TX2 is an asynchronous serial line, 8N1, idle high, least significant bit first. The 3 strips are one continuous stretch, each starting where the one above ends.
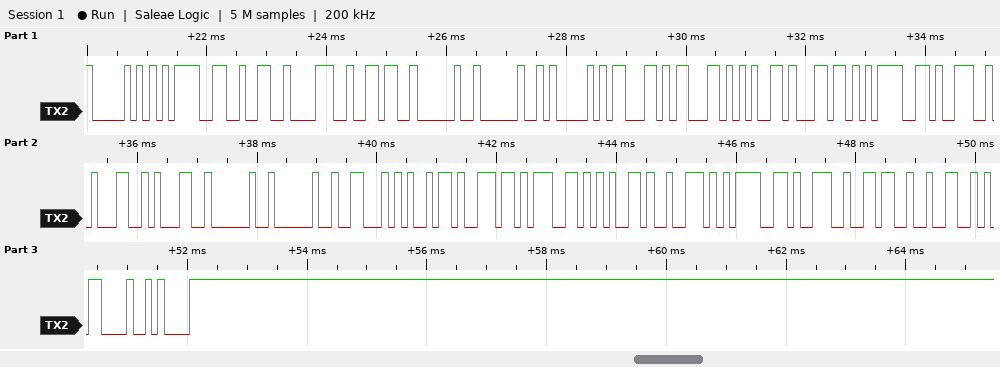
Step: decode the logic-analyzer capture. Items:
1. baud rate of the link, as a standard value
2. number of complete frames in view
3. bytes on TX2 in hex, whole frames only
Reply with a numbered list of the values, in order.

1. 9600 baud
2. 30
3. 50 3D 32 38 36 20 20 41 63 63 65 6C 3D 39 31 31 20 20 46 69 6E 67 65 72 3D 39 36 32 0D 0A
